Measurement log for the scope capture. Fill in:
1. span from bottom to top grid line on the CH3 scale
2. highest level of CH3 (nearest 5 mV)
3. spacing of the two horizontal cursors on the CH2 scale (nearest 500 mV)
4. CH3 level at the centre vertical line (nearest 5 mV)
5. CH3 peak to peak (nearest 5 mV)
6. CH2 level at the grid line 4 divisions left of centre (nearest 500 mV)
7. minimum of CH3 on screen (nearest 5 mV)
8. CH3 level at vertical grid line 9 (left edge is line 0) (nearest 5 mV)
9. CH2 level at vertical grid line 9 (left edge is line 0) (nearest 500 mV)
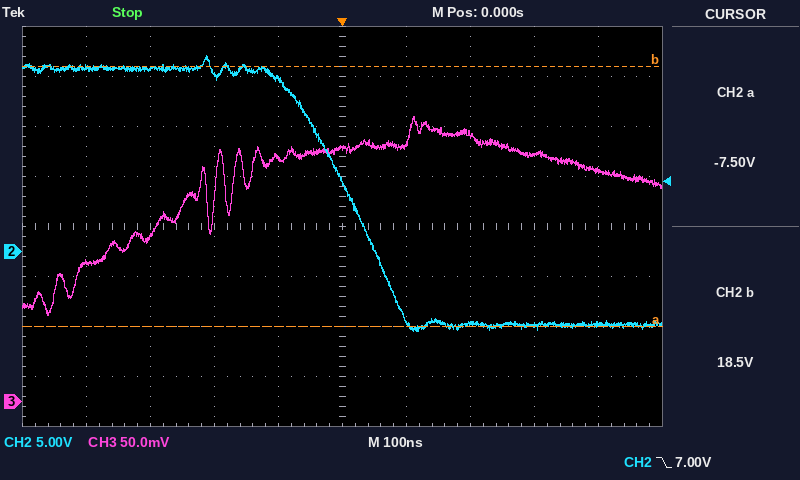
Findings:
400 mV
285 mV
26.0 V
255 mV
200 mV
18.5 V
85 mV
230 mV
-7.5 V
